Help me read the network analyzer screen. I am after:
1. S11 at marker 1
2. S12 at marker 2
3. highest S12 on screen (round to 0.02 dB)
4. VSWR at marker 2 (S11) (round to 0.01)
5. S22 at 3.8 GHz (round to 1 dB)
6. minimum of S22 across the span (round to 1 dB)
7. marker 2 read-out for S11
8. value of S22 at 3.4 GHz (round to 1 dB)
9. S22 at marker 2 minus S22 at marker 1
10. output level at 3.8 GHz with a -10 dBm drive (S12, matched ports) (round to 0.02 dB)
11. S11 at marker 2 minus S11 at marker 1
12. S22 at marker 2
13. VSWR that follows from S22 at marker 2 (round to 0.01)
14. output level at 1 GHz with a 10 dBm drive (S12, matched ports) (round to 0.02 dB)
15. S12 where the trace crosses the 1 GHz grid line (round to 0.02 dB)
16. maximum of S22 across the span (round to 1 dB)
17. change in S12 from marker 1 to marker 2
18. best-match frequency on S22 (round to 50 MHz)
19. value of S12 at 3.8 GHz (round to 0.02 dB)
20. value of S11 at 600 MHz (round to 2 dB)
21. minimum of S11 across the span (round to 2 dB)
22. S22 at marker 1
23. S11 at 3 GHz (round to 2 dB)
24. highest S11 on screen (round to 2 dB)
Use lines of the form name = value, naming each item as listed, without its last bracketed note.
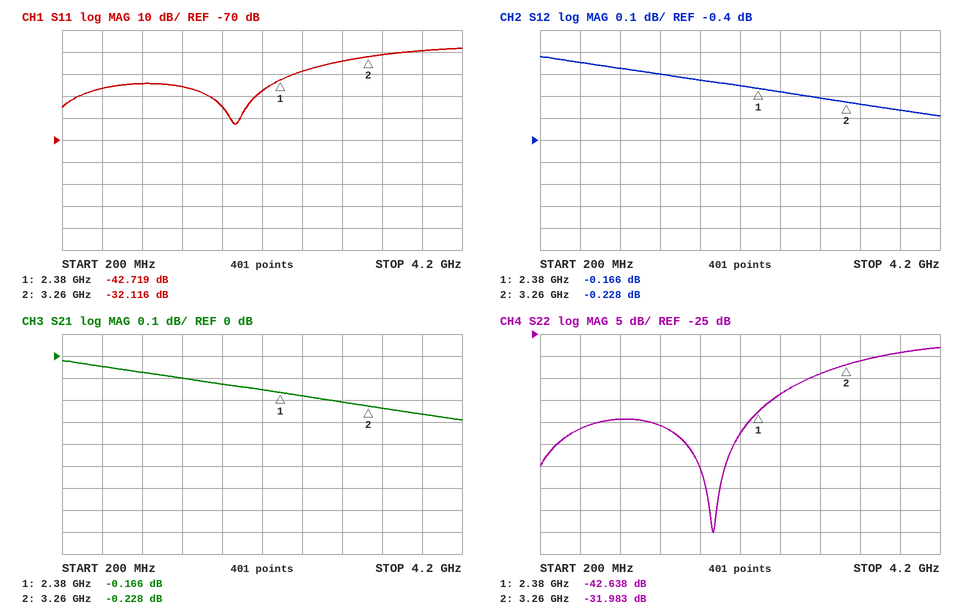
S11 at marker 1 = -42.719 dB
S12 at marker 2 = -0.228 dB
highest S12 on screen = -0.02 dB
VSWR at marker 2 (S11) = 1.05
S22 at 3.8 GHz = -29 dB
minimum of S22 across the span = -70 dB
marker 2 read-out for S11 = -32.116 dB
value of S22 at 3.4 GHz = -31 dB
S22 at marker 2 minus S22 at marker 1 = 10.655 dB
output level at 3.8 GHz with a -10 dBm drive (S12, matched ports) = -10.26 dBm
S11 at marker 2 minus S11 at marker 1 = 10.603 dB
S22 at marker 2 = -31.983 dB
VSWR that follows from S22 at marker 2 = 1.05
output level at 1 GHz with a 10 dBm drive (S12, matched ports) = 9.92 dBm
S12 where the trace crosses the 1 GHz grid line = -0.08 dB
maximum of S22 across the span = -28 dB
change in S12 from marker 1 to marker 2 = -0.062 dB
best-match frequency on S22 = 1.95 GHz
value of S12 at 3.8 GHz = -0.26 dB
value of S11 at 600 MHz = -46 dB
minimum of S11 across the span = -62 dB
S22 at marker 1 = -42.638 dB
S11 at 3 GHz = -34 dB
highest S11 on screen = -28 dB
